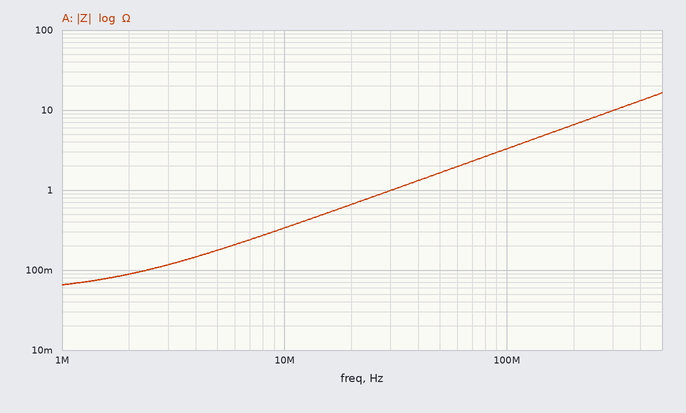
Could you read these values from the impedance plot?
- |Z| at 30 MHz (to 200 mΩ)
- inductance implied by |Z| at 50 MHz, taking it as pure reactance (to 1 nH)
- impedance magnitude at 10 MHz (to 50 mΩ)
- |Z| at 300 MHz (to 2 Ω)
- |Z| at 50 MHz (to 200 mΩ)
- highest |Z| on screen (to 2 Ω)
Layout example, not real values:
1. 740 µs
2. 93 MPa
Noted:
1. 1.0 Ω
2. 5 nH
3. 350 mΩ
4. 10 Ω
5. 1.6 Ω
6. 16 Ω
